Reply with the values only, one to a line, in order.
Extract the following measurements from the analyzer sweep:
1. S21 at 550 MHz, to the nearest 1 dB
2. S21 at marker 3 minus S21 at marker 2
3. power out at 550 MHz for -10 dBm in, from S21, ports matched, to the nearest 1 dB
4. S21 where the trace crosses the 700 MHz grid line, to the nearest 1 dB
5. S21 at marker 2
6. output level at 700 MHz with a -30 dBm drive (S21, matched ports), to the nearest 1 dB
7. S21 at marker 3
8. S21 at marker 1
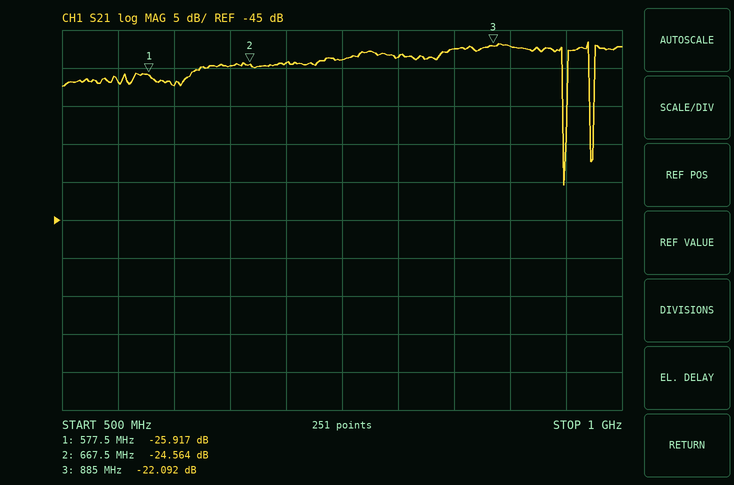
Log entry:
-27 dB
2.472 dB
-37 dBm
-24 dB
-24.564 dB
-54 dBm
-22.092 dB
-25.917 dB
